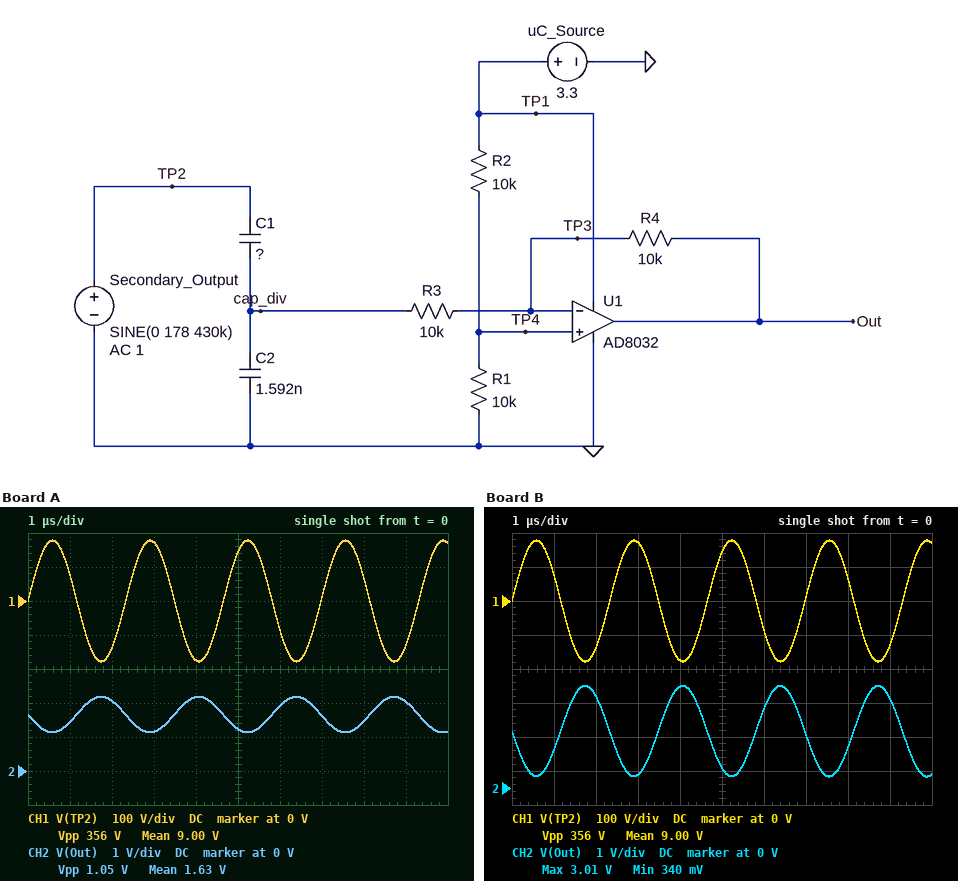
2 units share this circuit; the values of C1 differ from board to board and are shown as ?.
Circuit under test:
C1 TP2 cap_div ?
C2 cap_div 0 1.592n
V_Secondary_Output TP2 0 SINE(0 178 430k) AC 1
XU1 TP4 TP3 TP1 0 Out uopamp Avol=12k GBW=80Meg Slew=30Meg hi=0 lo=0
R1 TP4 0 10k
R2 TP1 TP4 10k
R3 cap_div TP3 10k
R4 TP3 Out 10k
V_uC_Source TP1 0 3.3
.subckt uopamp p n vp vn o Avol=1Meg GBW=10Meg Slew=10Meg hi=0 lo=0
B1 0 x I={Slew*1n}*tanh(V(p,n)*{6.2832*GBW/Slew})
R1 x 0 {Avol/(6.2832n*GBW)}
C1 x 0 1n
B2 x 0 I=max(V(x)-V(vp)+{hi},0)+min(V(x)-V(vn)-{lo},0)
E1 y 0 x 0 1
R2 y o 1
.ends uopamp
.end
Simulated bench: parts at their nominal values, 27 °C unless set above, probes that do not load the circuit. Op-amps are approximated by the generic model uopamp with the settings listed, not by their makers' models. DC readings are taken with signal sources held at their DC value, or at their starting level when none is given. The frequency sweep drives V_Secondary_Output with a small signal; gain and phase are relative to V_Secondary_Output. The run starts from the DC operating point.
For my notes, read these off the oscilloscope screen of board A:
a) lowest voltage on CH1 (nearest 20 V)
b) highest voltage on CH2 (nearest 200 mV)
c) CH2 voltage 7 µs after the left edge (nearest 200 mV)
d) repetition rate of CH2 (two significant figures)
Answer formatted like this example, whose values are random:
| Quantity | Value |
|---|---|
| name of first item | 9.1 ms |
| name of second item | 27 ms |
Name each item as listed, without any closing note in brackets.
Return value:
| Quantity | Value |
|---|---|
| lowest voltage on CH1 | -180 V |
| highest voltage on CH2 | 2.2 V |
| CH2 voltage 7 µs after the left edge | 1.6 V |
| repetition rate of CH2 | 430 kHz |
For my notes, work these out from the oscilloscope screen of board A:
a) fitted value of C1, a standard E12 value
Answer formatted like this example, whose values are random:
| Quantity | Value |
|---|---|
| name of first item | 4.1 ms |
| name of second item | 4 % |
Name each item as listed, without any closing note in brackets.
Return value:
| Quantity | Value |
|---|---|
| fitted value of C1, a standard E12 value | 4.7 pF |
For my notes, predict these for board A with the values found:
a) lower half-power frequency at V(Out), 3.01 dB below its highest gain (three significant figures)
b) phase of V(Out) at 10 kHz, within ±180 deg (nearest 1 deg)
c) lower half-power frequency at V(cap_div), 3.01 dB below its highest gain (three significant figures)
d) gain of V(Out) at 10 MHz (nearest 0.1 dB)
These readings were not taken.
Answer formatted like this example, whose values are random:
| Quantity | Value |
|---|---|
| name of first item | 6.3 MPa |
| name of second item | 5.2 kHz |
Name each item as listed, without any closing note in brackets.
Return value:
| Quantity | Value |
|---|---|
| lower half-power frequency at V(Out), 3.01 dB below its highest gain | 9.96 kHz |
| phase of V(Out) at 10 kHz, within ±180 deg | -135 deg |
| lower half-power frequency at V(cap_div), 3.01 dB below its highest gain | 9.97 kHz |
| gain of V(Out) at 10 MHz | -50.9 dB |
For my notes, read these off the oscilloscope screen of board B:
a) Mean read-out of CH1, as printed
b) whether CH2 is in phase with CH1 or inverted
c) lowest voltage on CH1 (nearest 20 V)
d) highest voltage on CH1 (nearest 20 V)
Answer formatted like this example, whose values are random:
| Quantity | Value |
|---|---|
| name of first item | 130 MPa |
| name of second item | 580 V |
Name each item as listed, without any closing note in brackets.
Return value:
| Quantity | Value |
|---|---|
| Mean read-out of CH1, as printed | 9.00 V |
| whether CH2 is in phase with CH1 or inverted | inverted |
| lowest voltage on CH1 | -180 V |
| highest voltage on CH1 | 180 V |
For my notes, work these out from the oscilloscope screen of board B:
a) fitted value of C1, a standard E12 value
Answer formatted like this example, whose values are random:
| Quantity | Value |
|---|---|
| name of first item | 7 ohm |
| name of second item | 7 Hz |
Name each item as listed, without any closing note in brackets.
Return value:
| Quantity | Value |
|---|---|
| fitted value of C1, a standard E12 value | 12 pF |
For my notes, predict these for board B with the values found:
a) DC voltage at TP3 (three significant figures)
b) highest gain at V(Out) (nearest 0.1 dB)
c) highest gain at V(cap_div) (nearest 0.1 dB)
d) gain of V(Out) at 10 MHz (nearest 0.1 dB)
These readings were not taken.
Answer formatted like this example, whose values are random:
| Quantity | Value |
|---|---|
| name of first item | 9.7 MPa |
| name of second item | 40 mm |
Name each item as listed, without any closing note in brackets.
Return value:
| Quantity | Value |
|---|---|
| DC voltage at TP3 | 1.65 V |
| highest gain at V(Out) | -42.5 dB |
| highest gain at V(cap_div) | -42.5 dB |
| gain of V(Out) at 10 MHz | -42.8 dB |
